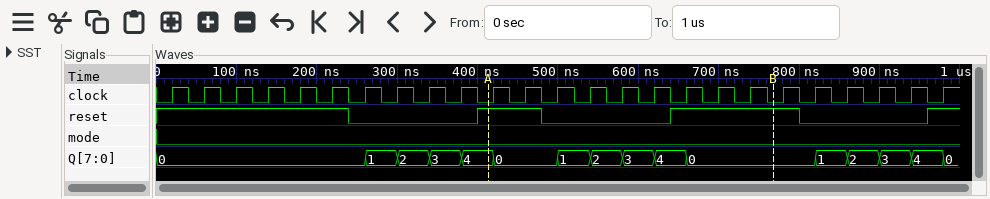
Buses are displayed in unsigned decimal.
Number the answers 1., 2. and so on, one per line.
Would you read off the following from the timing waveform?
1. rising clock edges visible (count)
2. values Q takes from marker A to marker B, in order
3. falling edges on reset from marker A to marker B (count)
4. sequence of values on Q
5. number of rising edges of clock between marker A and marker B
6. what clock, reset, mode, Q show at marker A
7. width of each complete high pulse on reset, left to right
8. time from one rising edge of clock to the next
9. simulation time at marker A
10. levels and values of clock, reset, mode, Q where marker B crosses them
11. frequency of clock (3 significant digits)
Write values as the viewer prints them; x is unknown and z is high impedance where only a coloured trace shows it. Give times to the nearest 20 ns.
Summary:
1. 25
2. 4, 0, 1, 2, 3, 4, 0
3. 1
4. 0, 1, 2, 3, 4, 0, 1, 2, 3, 4, 0, 1, 2, 3, 4, 0
5. 9
6. clock=0, reset=1, mode=0, Q=4
7. 80 ns, 160 ns
8. 40 ns
9. 420 ns
10. clock=0, reset=1, mode=0, Q=0
11. 25.0 MHz
